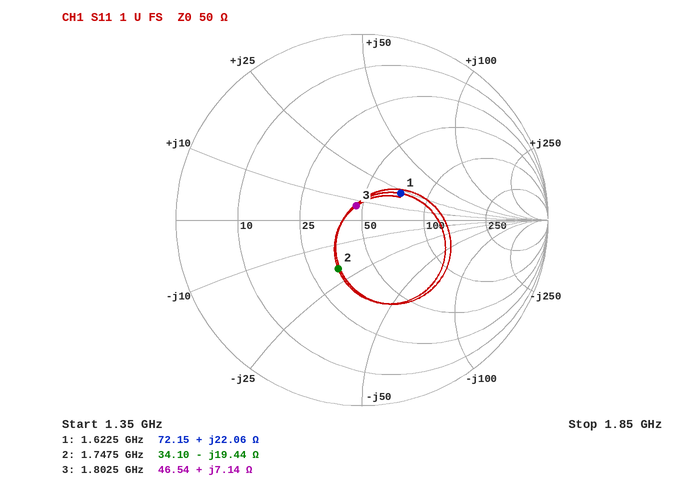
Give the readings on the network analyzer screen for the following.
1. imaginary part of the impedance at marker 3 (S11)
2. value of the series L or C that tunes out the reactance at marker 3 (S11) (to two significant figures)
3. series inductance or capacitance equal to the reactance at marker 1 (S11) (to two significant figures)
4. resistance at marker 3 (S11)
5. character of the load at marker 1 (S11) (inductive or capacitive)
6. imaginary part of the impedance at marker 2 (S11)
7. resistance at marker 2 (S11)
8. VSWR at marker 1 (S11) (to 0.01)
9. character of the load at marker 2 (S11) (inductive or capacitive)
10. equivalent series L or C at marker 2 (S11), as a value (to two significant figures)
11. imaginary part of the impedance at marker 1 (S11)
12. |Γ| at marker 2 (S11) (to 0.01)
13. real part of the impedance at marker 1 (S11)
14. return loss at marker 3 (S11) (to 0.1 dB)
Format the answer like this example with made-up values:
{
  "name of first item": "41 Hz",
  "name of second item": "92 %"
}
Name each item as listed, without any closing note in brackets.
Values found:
{
  "imaginary part of the impedance at marker 3": "+7.14 Ω",
  "value of the series L or C that tunes out the reactance at marker 3 (S11)": "12 pF",
  "series inductance or capacitance equal to the reactance at marker 1 (S11)": "2.2 nH",
  "resistance at marker 3": "46.54 Ω",
  "character of the load at marker 1 (S11)": "inductive",
  "imaginary part of the impedance at marker 2": "-19.44 Ω",
  "resistance at marker 2": "34.10 Ω",
  "VSWR at marker 1 (S11)": "1.67",
  "character of the load at marker 2 (S11)": "capacitive",
  "equivalent series L or C at marker 2 (S11), as a value": "4.7 pF",
  "imaginary part of the impedance at marker 1": "+22.06 Ω",
  "|Γ| at marker 2 (S11)": "0.29",
  "real part of the impedance at marker 1": "72.15 Ω",
  "return loss at marker 3 (S11)": "21.7 dB"
}
